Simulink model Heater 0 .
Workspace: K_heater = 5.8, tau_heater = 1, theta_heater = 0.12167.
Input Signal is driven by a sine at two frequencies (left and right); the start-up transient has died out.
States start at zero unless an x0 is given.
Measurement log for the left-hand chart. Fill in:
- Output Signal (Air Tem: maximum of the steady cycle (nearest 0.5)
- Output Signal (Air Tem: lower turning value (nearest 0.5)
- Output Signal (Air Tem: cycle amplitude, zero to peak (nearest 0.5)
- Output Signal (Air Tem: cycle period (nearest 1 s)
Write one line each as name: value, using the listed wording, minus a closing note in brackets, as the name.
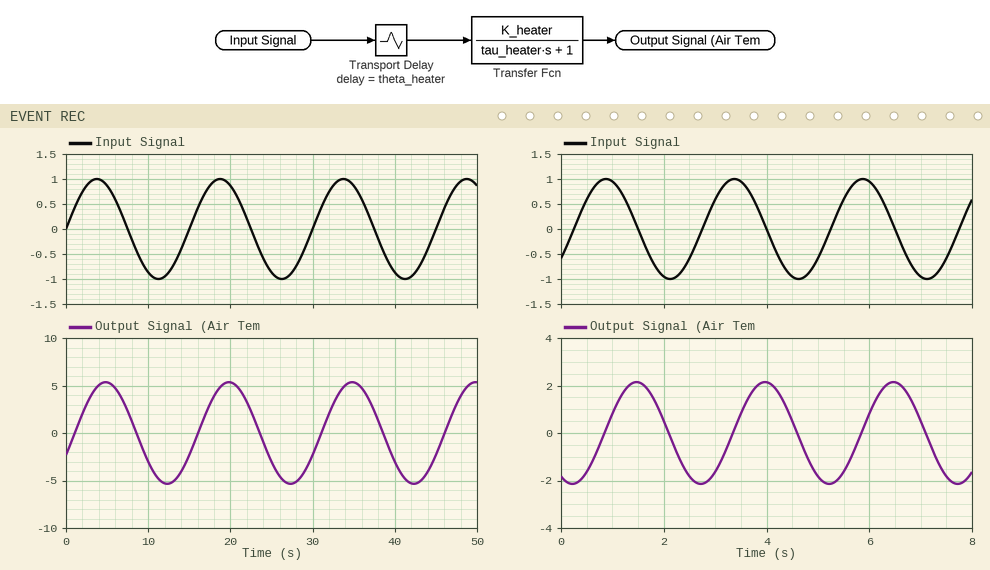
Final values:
Output Signal (Air Tem: maximum of the steady cycle: 5.5
Output Signal (Air Tem: lower turning value: -5.5
Output Signal (Air Tem: cycle amplitude, zero to peak: 5.5
Output Signal (Air Tem: cycle period: 15 s
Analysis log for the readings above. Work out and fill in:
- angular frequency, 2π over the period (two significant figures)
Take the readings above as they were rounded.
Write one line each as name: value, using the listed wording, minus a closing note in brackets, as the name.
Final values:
angular frequency, 2π over the period: 0.42 rad/s
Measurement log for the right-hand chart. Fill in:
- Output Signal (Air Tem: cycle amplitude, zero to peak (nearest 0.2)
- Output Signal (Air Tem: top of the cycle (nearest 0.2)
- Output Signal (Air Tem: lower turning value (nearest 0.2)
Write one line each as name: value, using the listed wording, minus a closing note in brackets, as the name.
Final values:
Output Signal (Air Tem: cycle amplitude, zero to peak: 2.2
Output Signal (Air Tem: top of the cycle: 2.2
Output Signal (Air Tem: lower turning value: -2.2
